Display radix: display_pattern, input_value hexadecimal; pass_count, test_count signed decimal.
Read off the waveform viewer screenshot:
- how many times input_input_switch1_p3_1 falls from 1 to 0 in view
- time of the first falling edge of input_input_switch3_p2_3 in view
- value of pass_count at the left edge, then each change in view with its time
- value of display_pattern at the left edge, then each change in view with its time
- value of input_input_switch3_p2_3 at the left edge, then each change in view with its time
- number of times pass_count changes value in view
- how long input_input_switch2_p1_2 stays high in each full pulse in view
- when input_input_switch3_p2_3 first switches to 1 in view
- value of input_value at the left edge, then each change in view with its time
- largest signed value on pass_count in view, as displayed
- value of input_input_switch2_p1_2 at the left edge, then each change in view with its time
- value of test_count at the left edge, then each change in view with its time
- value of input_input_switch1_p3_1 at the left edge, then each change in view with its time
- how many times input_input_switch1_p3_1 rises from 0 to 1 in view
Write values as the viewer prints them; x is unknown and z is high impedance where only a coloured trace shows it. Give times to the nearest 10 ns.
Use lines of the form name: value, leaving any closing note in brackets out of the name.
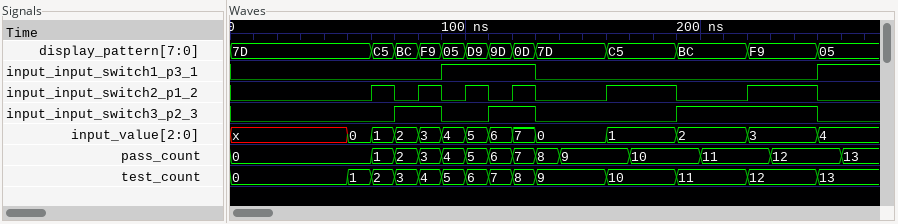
how many times input_input_switch1_p3_1 falls from 1 to 0 in view: 1
time of the first falling edge of input_input_switch3_p2_3 in view: 90 ns
value of pass_count at the left edge, then each change in view with its time: 0, 1 at 60 ns, 2 at 70 ns, 3 at 80 ns, 4 at 90 ns, 5 at 100 ns, 6 at 110 ns, 7 at 120 ns, 8 at 130 ns, 9 at 140 ns, 10 at 170 ns, 11 at 200 ns, 12 at 230 ns, 13 at 260 ns
value of display_pattern at the left edge, then each change in view with its time: 7D, C5 at 60 ns, BC at 70 ns, F9 at 80 ns, 05 at 90 ns, D9 at 100 ns, 9D at 110 ns, 0D at 120 ns, 7D at 130 ns, C5 at 160 ns, BC at 190 ns, F9 at 220 ns, 05 at 250 ns
value of input_input_switch3_p2_3 at the left edge, then each change in view with its time: 0, 1 at 70 ns, 0 at 90 ns, 1 at 110 ns, 0 at 130 ns, 1 at 190 ns, 0 at 250 ns
number of times pass_count changes value in view: 13
how long input_input_switch2_p1_2 stays high in each full pulse in view: 10 ns, 10 ns, 10 ns, 10 ns, 30 ns, 30 ns
when input_input_switch3_p2_3 first switches to 1 in view: 70 ns
value of input_value at the left edge, then each change in view with its time: x, 0 at 50 ns, 1 at 60 ns, 2 at 70 ns, 3 at 80 ns, 4 at 90 ns, 5 at 100 ns, 6 at 110 ns, 7 at 120 ns, 0 at 130 ns, 1 at 160 ns, 2 at 190 ns, 3 at 220 ns, 4 at 250 ns
largest signed value on pass_count in view, as displayed: 13
value of input_input_switch2_p1_2 at the left edge, then each change in view with its time: 0, 1 at 60 ns, 0 at 70 ns, 1 at 80 ns, 0 at 90 ns, 1 at 100 ns, 0 at 110 ns, 1 at 120 ns, 0 at 130 ns, 1 at 160 ns, 0 at 190 ns, 1 at 220 ns, 0 at 250 ns
value of test_count at the left edge, then each change in view with its time: 0, 1 at 50 ns, 2 at 60 ns, 3 at 70 ns, 4 at 80 ns, 5 at 90 ns, 6 at 100 ns, 7 at 110 ns, 8 at 120 ns, 9 at 130 ns, 10 at 160 ns, 11 at 190 ns, 12 at 220 ns, 13 at 250 ns
value of input_input_switch1_p3_1 at the left edge, then each change in view with its time: 0, 1 at 90 ns, 0 at 130 ns, 1 at 250 ns
how many times input_input_switch1_p3_1 rises from 0 to 1 in view: 2
